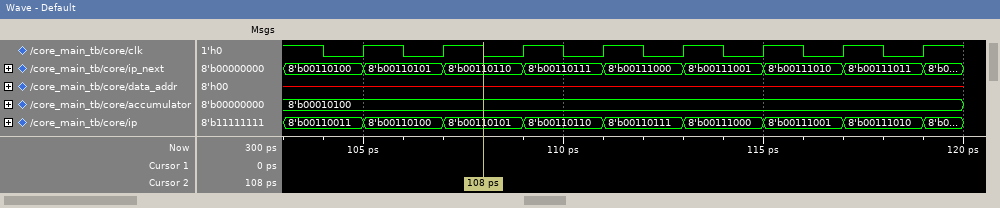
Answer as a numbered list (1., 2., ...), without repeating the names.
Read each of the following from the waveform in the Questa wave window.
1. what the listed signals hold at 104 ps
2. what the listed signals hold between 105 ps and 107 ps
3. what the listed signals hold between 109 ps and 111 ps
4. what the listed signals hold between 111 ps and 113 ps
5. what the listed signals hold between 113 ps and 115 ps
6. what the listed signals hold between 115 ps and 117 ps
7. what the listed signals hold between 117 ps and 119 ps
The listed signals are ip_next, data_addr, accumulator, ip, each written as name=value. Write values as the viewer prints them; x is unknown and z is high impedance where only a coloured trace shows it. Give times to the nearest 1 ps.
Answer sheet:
1. ip_next=8'b00110100, data_addr=x, accumulator=8'b00010100, ip=8'b00110011
2. ip_next=8'b00110101, data_addr=x, accumulator=8'b00010100, ip=8'b00110100
3. ip_next=8'b00110111, data_addr=x, accumulator=8'b00010100, ip=8'b00110110
4. ip_next=8'b00111000, data_addr=x, accumulator=8'b00010100, ip=8'b00110111
5. ip_next=8'b00111001, data_addr=x, accumulator=8'b00010100, ip=8'b00111000
6. ip_next=8'b00111010, data_addr=x, accumulator=8'b00010100, ip=8'b00111001
7. ip_next=8'b00111011, data_addr=x, accumulator=8'b00010100, ip=8'b00111010
